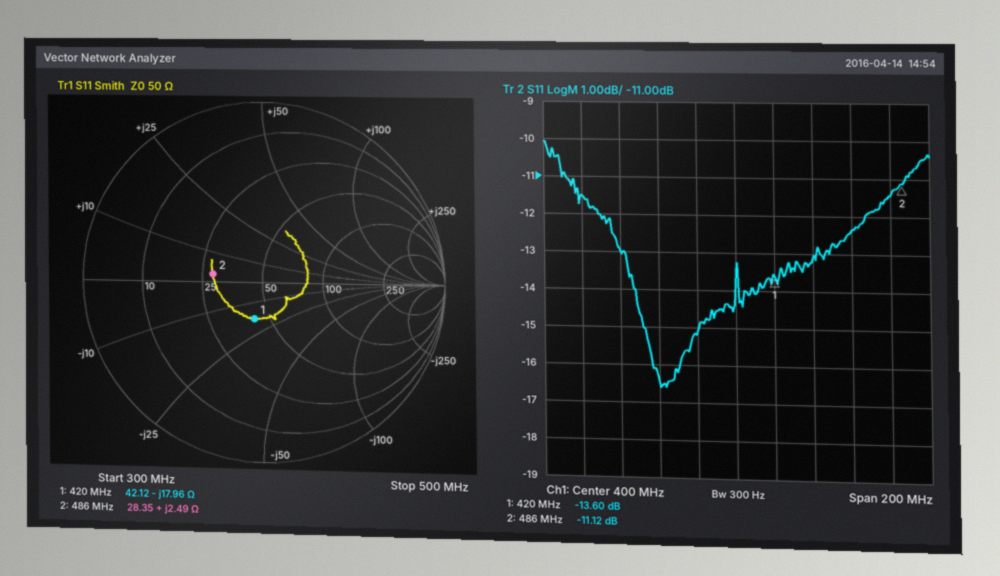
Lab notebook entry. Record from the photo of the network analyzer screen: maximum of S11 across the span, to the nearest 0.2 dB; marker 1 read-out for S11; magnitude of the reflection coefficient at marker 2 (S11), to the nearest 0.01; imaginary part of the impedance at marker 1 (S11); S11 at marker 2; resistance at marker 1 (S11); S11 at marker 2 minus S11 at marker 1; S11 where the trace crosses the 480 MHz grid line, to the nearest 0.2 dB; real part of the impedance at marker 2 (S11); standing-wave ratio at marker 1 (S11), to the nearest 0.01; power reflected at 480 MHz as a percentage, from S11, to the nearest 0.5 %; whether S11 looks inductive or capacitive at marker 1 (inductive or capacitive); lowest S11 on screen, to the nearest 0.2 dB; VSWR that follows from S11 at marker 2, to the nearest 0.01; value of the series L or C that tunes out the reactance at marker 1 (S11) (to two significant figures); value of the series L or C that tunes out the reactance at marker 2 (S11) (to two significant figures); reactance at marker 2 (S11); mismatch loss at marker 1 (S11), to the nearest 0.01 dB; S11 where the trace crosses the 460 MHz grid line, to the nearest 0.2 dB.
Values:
-10.0 dB
-13.60 dB
0.28
-17.96 Ω
-11.12 dB
42.12 Ω
2.48 dB
-11.4 dB
28.35 Ω
1.53
7.0 %
capacitive
-16.6 dB
1.77
6.8 nH
130 pF
+2.49 Ω
0.19 dB
-12.4 dB
